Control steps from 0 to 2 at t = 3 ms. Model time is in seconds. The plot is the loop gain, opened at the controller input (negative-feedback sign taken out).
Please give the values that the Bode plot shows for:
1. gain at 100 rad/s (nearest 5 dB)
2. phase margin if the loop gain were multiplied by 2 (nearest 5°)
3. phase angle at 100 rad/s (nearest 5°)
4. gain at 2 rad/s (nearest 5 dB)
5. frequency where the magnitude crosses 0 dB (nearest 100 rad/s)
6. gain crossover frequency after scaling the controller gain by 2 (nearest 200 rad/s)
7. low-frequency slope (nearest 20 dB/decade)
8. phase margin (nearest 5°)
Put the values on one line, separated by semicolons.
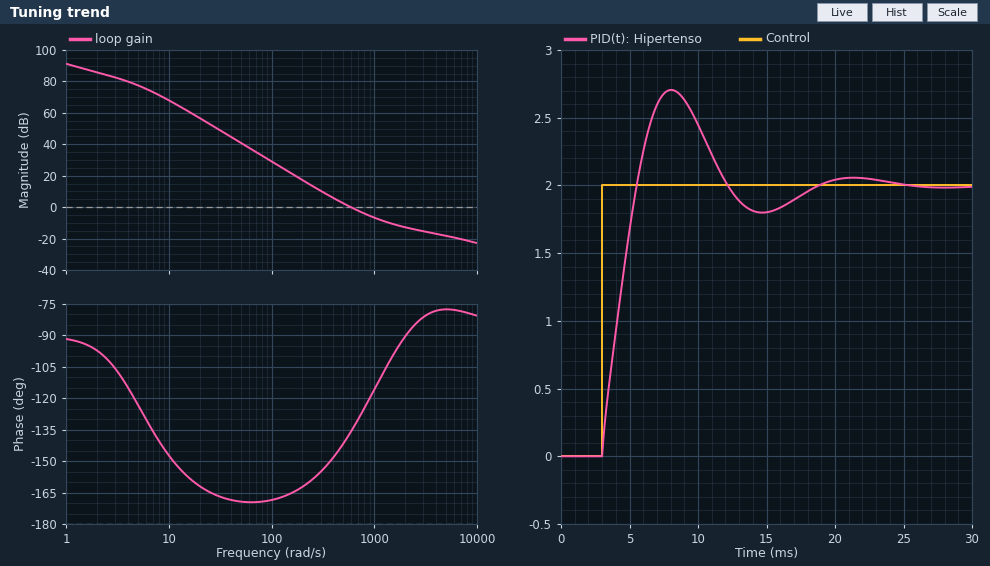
30 dB; 60°; -170°; 85 dB; 600 rad/s; 1000 rad/s; -20 dB/decade; 45°
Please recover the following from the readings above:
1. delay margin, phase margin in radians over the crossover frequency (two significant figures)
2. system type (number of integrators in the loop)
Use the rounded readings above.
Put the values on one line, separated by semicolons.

0.0013 s; 1
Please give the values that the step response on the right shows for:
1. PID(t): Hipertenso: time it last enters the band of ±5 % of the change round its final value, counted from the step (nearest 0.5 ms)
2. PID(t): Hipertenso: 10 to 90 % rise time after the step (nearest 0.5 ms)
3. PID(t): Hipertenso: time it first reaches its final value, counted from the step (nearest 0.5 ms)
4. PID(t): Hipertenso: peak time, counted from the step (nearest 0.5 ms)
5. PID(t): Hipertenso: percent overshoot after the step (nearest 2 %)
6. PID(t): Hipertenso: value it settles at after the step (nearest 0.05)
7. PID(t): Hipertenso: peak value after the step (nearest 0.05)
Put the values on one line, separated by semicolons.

14.0 ms; 2.0 ms; 2.5 ms; 5.0 ms; 36 %; 2.00; 2.70
